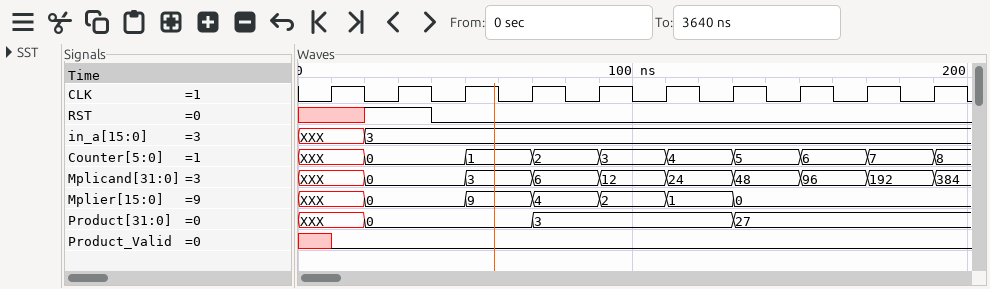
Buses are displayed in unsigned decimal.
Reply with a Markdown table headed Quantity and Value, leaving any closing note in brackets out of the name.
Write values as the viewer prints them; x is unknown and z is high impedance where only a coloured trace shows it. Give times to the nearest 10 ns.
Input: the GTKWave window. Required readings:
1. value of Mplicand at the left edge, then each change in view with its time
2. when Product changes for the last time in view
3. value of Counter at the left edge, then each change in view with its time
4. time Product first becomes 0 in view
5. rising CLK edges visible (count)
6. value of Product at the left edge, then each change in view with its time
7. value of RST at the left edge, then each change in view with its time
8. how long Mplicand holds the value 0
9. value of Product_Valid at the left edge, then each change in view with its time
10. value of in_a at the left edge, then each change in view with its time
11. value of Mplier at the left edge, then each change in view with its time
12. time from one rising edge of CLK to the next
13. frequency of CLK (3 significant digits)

| Quantity | Value |
|---|---|
| value of Mplicand at the left edge, then each change in view with its time | XXX, 0 at 20 ns, 3 at 50 ns, 6 at 70 ns, 12 at 90 ns, 24 at 110 ns, 48 at 130 ns, 96 at 150 ns, 192 at 170 ns, 384 at 190 ns |
| when Product changes for the last time in view | 130 ns |
| value of Counter at the left edge, then each change in view with its time | XXX, 0 at 20 ns, 1 at 50 ns, 2 at 70 ns, 3 at 90 ns, 4 at 110 ns, 5 at 130 ns, 6 at 150 ns, 7 at 170 ns, 8 at 190 ns |
| time Product first becomes 0 in view | 20 ns |
| rising CLK edges visible | 10 |
| value of Product at the left edge, then each change in view with its time | XXX, 0 at 20 ns, 3 at 70 ns, 27 at 130 ns |
| value of RST at the left edge, then each change in view with its time | x, 1 at 20 ns, 0 at 40 ns |
| how long Mplicand holds the value 0 | 30 ns |
| value of Product_Valid at the left edge, then each change in view with its time | x, 0 at 10 ns |
| value of in_a at the left edge, then each change in view with its time | XXX, 3 at 20 ns |
| value of Mplier at the left edge, then each change in view with its time | XXX, 0 at 20 ns, 9 at 50 ns, 4 at 70 ns, 2 at 90 ns, 1 at 110 ns, 0 at 130 ns |
| time from one rising edge of CLK to the next | 20 ns |
| frequency of CLK | 50.0 MHz |
